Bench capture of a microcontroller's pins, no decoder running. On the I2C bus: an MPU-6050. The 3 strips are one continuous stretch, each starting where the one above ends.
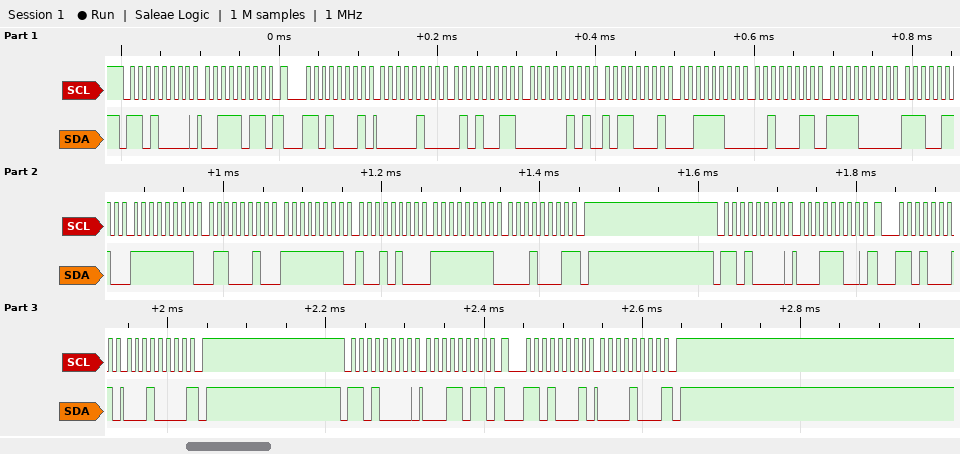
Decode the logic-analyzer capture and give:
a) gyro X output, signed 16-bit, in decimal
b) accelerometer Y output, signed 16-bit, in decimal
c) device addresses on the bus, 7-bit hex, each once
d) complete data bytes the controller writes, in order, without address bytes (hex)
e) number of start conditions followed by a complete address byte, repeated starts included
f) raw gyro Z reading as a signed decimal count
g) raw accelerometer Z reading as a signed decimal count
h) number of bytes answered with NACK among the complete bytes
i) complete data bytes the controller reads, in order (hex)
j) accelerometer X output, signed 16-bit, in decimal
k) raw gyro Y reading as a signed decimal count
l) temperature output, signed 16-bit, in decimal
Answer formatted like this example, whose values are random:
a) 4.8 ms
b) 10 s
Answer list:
a) -158
b) 1457
c) 0x68
d) 3B 1C 1B
e) 6
f) -239
g) 15395
h) 3
i) 04 53 05 B1 3C 23 F0 E6 FF 62 FF 94 FF 11 10 08
j) 1107
k) -108
l) -3866
